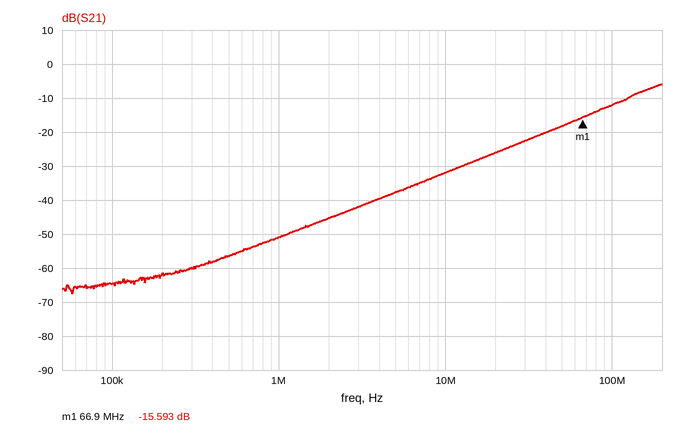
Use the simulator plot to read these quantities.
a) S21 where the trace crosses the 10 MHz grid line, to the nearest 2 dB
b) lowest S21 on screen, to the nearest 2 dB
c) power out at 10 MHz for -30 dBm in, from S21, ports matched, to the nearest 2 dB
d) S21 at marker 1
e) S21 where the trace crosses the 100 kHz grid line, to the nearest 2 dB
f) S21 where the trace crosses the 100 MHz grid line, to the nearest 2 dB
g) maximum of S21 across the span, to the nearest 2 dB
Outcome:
-32 dB
-68 dB
-62 dBm
-15.593 dB
-64 dB
-12 dB
-6 dB
